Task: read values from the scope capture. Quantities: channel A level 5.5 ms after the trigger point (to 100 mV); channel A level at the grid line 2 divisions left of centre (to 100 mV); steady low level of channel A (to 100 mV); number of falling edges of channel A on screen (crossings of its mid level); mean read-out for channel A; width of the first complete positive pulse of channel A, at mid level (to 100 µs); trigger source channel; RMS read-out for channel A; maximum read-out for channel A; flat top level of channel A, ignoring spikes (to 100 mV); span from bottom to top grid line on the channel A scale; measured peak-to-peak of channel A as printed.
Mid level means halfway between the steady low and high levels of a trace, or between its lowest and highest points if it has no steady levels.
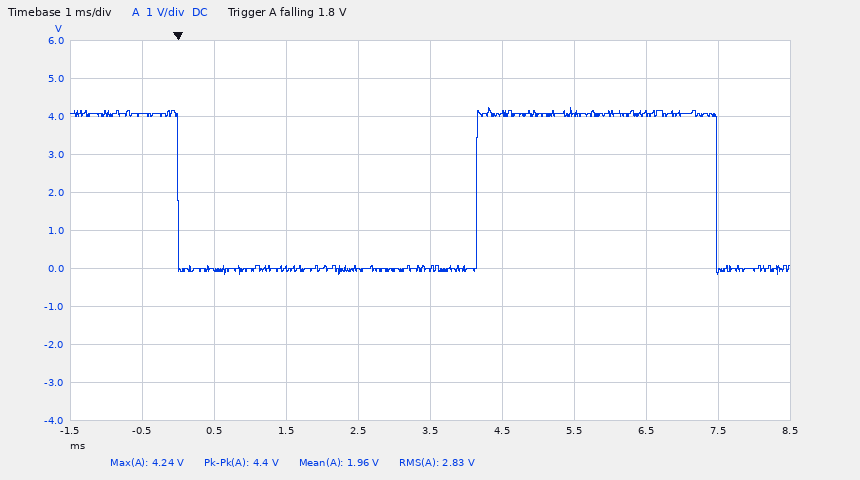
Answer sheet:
4.1 V
0.0 V
0.0 V
2
1.96 V
3.3 ms
channel A
2.83 V
4.24 V
4.1 V
10 V
4.4 V
